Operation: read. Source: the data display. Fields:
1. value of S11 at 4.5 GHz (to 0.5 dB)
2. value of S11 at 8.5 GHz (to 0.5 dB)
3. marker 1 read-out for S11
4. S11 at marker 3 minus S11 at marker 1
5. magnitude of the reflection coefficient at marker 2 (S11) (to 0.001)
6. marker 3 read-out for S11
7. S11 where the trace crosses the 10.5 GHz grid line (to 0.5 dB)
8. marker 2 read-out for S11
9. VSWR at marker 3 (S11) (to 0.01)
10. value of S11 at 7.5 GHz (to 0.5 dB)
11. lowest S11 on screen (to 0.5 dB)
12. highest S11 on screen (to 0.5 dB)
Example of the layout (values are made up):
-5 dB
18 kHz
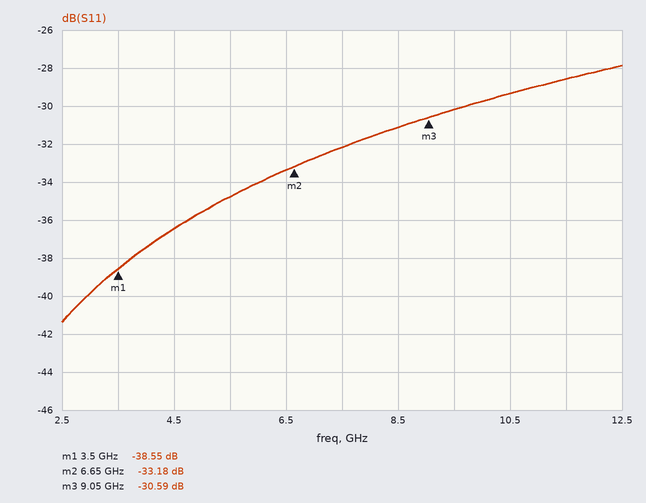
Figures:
-36.5 dB
-31.0 dB
-38.55 dB
7.96 dB
0.022
-30.59 dB
-29.5 dB
-33.18 dB
1.06
-32.0 dB
-41.5 dB
-28.0 dB
